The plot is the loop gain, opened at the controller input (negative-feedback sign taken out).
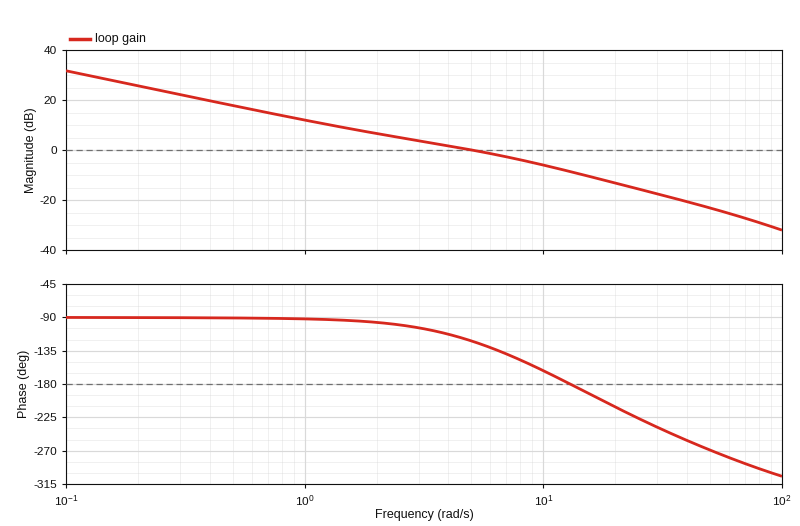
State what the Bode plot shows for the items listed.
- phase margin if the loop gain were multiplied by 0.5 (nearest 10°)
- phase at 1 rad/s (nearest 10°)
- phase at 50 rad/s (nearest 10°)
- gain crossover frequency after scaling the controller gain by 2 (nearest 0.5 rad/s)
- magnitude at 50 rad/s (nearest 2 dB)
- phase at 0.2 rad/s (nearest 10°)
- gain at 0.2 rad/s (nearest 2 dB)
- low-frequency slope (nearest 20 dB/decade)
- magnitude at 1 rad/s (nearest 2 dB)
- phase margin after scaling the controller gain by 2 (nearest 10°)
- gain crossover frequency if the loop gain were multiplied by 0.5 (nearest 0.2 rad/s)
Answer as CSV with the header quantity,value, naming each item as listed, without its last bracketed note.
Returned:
quantity,value
phase margin if the loop gain were multiplied by 0.5,80°
phase at 1 rad/s,-90°
phase at 50 rad/s,-270°
gain crossover frequency after scaling the controller gain by 2,10.0 rad/s
magnitude at 50 rad/s,-24 dB
phase at 0.2 rad/s,-90°
gain at 0.2 rad/s,26 dB
low-frequency slope,-20 dB/decade
magnitude at 1 rad/s,12 dB
phase margin after scaling the controller gain by 2,20°
gain crossover frequency if the loop gain were multiplied by 0.5,2.2 rad/s
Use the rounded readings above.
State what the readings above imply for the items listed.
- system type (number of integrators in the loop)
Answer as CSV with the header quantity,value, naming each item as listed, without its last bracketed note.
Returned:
quantity,value
system type,1
